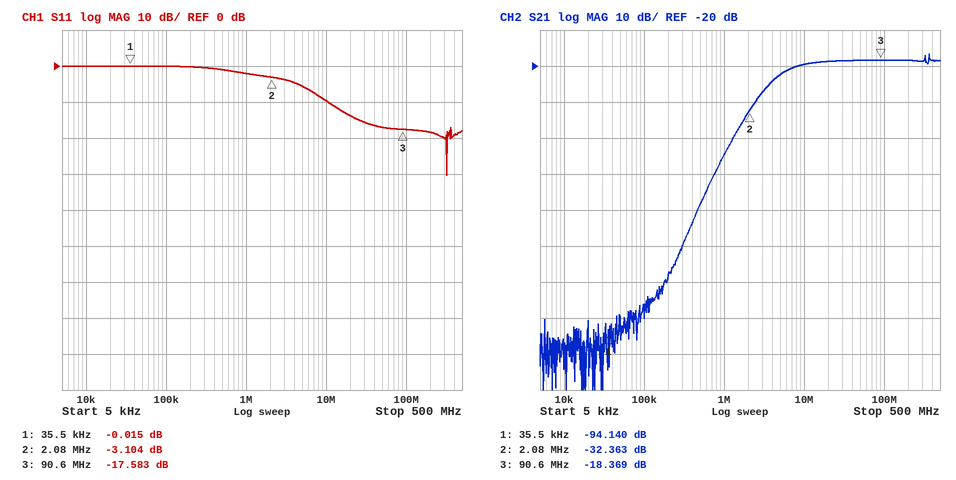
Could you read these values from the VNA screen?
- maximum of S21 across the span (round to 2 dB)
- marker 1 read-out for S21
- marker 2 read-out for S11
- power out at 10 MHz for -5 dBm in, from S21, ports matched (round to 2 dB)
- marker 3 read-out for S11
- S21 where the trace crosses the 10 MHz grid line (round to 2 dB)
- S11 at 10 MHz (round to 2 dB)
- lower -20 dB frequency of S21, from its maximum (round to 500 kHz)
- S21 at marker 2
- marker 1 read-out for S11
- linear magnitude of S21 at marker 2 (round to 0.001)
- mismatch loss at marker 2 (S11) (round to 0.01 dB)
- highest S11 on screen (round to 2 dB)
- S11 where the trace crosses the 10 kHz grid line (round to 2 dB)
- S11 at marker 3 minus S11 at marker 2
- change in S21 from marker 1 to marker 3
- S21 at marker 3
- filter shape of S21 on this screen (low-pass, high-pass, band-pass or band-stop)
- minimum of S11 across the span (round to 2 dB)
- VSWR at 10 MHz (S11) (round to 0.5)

-16 dB
-94.140 dB
-3.104 dB
-24 dBm
-17.583 dB
-20 dB
-10 dB
1.5 MHz
-32.363 dB
-0.015 dB
0.024
2.92 dB
0 dB
0 dB
-14.479 dB
75.771 dB
-18.369 dB
high-pass
-30 dB
2.0
